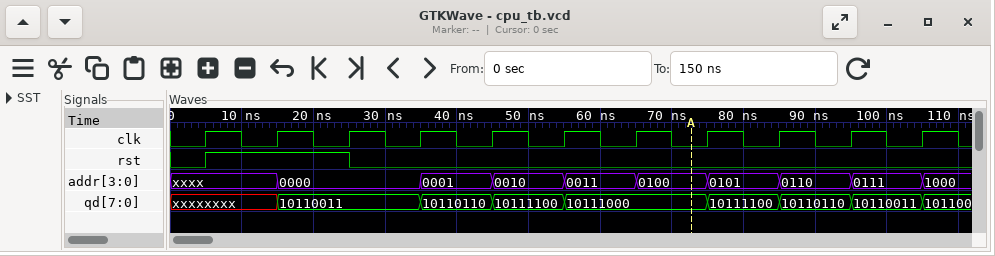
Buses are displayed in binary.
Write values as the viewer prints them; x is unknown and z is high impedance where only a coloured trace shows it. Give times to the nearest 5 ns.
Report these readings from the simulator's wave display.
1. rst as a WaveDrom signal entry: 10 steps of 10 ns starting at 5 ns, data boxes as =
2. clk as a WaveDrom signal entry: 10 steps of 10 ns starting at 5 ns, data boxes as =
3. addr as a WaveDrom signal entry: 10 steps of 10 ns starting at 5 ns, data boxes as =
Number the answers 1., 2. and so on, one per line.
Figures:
1. {name: 'rst', wave: '1.0.......'}
2. {name: 'clk', wave: 'p.........'}
3. {name: 'addr', wave: 'x=.=======', data: '0000 0001 0010 0011 0100 0101 0110 0111'}
